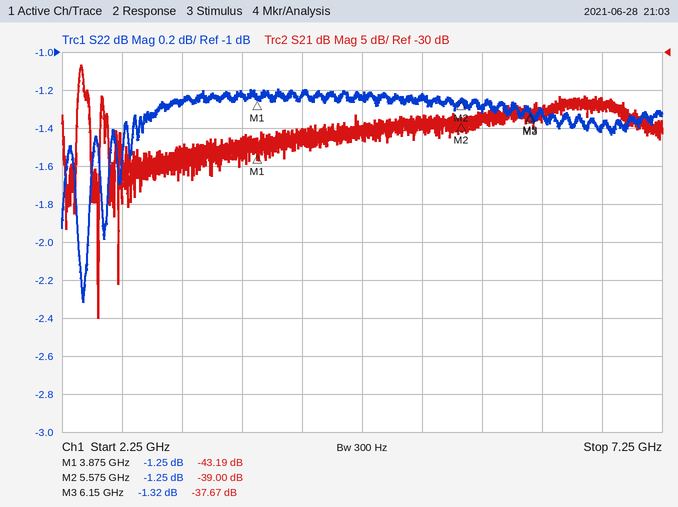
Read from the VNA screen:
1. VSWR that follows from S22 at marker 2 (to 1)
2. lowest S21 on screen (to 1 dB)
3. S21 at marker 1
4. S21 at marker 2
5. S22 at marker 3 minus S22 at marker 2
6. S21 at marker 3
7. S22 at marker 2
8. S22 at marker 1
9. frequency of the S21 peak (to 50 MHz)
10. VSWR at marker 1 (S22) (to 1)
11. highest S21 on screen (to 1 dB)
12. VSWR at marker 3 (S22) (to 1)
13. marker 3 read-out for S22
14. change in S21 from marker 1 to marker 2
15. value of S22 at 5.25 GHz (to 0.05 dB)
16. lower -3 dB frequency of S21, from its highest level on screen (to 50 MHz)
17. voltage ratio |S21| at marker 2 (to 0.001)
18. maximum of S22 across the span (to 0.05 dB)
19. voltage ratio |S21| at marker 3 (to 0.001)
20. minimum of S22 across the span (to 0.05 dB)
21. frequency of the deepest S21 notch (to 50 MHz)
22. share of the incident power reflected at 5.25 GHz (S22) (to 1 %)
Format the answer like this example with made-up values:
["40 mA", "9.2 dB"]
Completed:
["14", "-65 dB", "-43.19 dB", "-39.00 dB", "-0.07 dB", "-37.67 dB", "-1.25 dB", "-1.25 dB", "2.40 GHz", "14", "-32 dB", "13", "-1.32 dB", "4.19 dB", "-1.25 dB", "2.40 GHz", "0.011", "-1.20 dB", "0.013", "-2.30 dB", "2.55 GHz", "75 %"]
